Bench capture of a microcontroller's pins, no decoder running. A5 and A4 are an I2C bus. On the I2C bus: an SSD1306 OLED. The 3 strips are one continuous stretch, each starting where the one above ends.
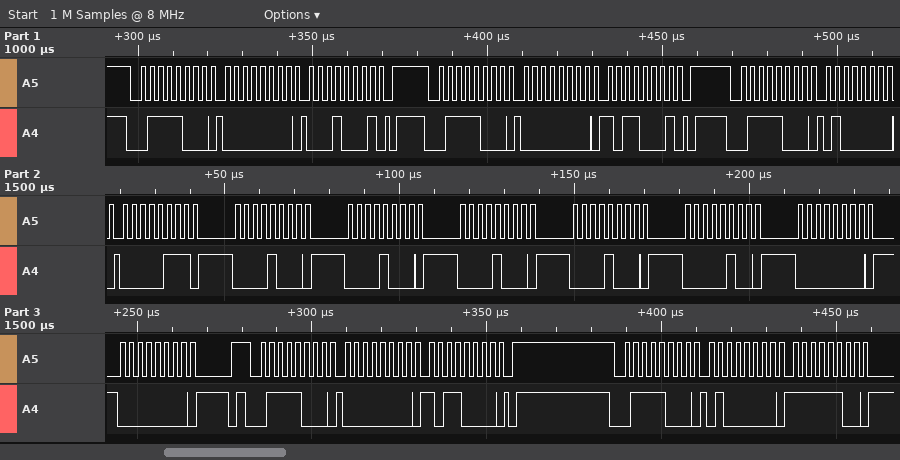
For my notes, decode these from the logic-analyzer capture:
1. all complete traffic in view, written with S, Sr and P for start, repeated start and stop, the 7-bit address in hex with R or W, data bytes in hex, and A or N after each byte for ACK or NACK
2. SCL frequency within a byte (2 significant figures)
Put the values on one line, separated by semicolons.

S 3CW A 00 A 11 A P S 3CW A 00 A B1 A P S 3CW A 40 A 07 A 08 A 08 A 08 A 08 A 04 A 00 A 00 A P S 3CW A 00 A B0 A P S 3CW A 40 A FC A; 400 kHz
